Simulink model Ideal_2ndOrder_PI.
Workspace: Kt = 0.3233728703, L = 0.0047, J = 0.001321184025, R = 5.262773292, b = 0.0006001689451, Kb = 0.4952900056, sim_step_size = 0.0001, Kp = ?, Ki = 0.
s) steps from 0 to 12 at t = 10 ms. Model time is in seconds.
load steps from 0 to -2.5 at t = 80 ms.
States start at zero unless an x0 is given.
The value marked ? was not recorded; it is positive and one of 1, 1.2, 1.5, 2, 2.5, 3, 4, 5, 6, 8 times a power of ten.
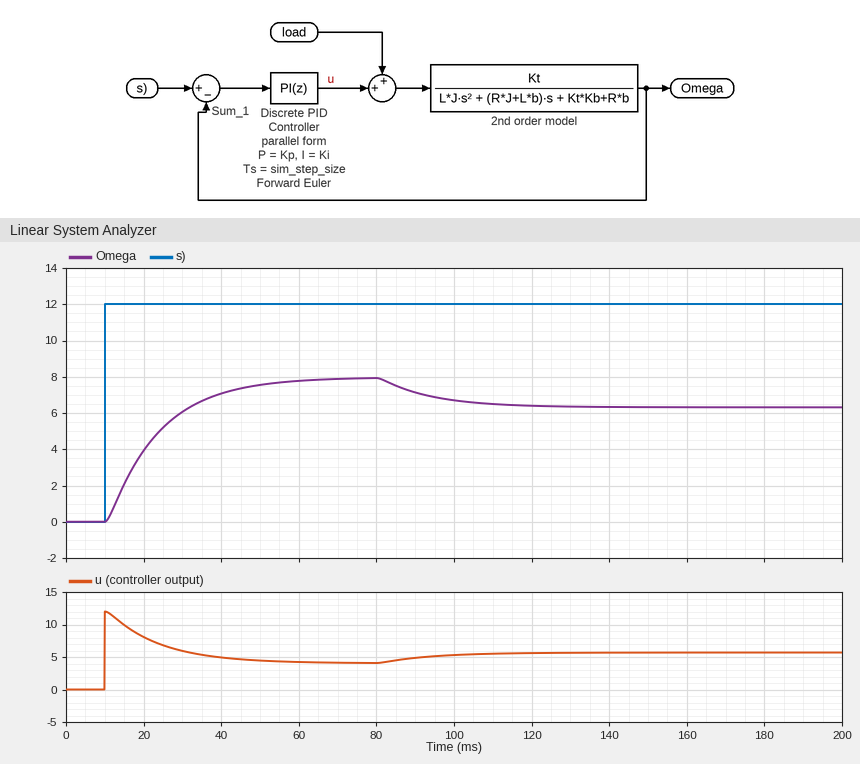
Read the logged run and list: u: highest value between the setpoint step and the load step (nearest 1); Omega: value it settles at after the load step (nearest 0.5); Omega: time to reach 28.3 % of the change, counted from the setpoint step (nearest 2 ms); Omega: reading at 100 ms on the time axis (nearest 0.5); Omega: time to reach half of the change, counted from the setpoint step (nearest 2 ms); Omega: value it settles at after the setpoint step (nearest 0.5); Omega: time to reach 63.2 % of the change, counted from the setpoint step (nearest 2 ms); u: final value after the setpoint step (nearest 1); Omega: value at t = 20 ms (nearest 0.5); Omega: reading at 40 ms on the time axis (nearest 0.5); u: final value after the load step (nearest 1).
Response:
12
6.5
6 ms
6.5
10 ms
8.0
14 ms
4
4.0
7.0
6
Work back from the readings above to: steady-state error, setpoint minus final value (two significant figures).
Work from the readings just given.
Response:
4.0
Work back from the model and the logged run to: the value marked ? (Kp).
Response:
1
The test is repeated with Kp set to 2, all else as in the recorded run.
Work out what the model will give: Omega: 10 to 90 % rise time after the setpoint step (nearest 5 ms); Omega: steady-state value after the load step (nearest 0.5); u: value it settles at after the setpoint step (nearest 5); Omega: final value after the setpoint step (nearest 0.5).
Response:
15 ms
8.5
5
9.5
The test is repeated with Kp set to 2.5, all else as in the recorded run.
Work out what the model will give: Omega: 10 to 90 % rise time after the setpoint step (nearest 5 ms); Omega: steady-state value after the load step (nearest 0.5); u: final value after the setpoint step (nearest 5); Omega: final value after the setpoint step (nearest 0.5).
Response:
15 ms
9.0
5
10.0
